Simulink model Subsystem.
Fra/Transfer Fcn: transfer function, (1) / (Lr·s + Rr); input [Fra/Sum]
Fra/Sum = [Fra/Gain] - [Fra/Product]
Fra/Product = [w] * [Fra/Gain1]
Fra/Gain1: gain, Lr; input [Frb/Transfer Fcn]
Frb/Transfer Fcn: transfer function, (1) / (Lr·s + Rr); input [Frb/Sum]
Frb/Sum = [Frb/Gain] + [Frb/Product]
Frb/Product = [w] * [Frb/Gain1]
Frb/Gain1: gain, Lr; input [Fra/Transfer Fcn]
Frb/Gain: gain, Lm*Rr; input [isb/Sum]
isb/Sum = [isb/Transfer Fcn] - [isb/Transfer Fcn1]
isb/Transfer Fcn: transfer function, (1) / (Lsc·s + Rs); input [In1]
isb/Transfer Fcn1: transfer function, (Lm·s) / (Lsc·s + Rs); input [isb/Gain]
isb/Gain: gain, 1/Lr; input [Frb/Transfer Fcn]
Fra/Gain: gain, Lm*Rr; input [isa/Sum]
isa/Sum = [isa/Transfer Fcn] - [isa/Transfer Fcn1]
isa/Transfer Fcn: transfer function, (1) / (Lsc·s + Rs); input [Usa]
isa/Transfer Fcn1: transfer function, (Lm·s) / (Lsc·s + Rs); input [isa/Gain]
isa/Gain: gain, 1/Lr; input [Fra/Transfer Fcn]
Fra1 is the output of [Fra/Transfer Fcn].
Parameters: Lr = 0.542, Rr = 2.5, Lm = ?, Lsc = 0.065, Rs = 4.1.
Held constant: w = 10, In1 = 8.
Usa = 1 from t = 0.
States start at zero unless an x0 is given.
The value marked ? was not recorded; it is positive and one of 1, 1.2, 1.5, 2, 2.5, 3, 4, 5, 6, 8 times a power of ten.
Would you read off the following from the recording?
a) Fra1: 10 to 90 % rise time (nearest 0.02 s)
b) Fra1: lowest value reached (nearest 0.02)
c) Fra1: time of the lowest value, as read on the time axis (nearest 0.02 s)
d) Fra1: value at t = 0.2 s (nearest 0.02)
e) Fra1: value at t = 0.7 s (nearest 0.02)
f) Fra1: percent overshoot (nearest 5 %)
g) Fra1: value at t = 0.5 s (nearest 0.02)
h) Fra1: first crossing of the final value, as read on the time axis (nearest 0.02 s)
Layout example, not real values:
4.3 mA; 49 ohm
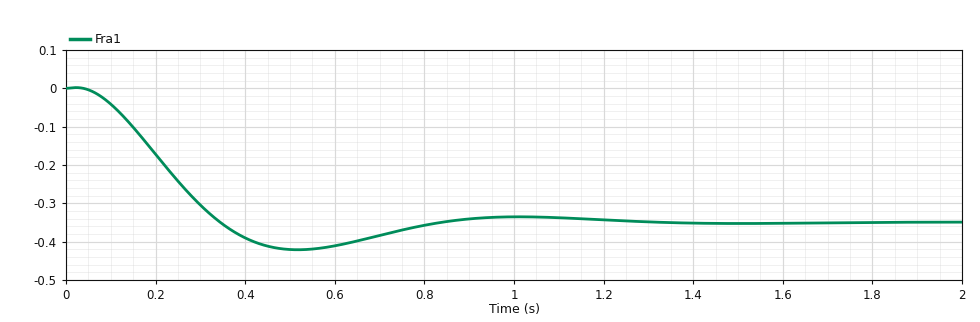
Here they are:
0.22 s; -0.42; 0.52 s; -0.18; -0.38; 20 %; -0.42; 0.34 s
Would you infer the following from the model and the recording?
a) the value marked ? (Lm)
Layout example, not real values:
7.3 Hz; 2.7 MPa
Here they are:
0.5
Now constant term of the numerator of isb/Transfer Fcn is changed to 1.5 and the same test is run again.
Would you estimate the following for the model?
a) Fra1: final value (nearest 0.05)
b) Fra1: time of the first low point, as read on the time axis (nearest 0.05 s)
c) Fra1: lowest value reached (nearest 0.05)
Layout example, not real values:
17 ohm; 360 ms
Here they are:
-0.55; 0.50 s; -0.65
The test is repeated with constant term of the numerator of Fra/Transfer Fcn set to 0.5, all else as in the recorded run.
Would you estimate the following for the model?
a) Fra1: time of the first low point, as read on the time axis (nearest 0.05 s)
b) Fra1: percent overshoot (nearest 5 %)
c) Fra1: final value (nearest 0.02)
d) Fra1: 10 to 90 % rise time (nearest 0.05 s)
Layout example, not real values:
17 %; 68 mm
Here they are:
0.65 s; 10 %; -0.30; 0.30 s
